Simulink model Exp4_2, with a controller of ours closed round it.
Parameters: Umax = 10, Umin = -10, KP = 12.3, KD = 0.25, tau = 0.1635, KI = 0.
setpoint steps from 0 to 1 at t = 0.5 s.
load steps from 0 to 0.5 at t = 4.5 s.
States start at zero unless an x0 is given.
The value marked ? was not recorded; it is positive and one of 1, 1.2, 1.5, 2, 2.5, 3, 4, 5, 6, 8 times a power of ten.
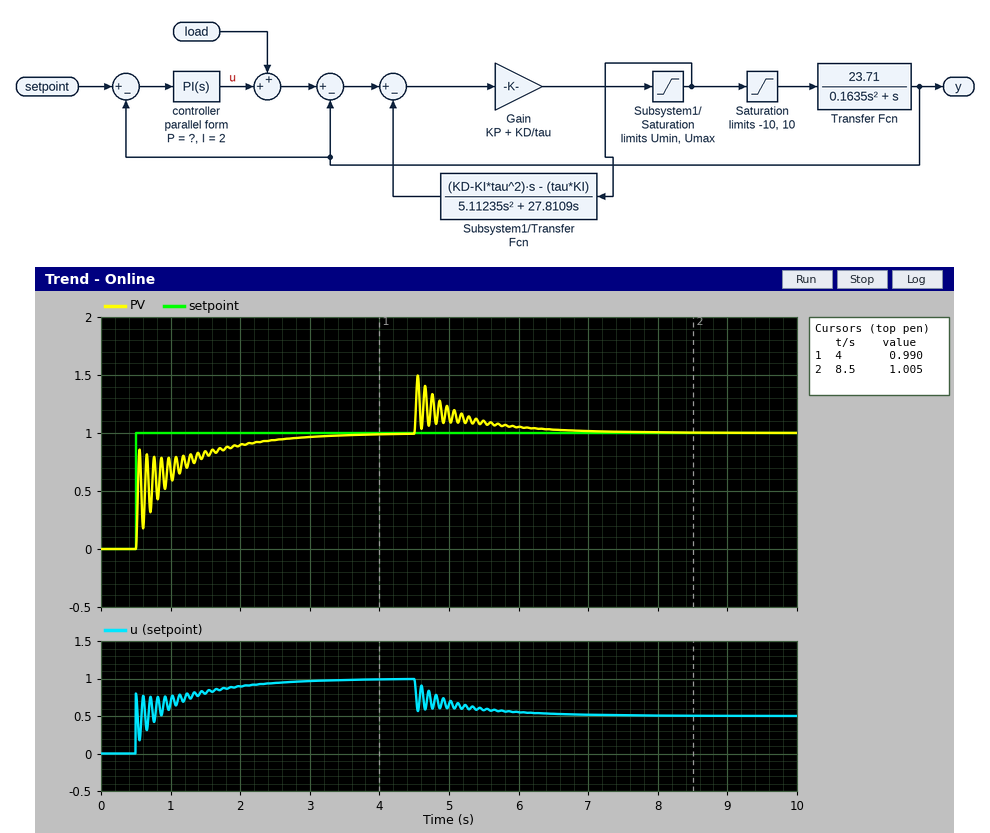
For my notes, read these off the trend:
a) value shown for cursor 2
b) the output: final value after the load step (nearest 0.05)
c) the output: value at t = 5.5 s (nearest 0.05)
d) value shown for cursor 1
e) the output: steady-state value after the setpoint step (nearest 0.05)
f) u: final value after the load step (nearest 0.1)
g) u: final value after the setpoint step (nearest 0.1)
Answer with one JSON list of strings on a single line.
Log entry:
["1.005", "1.00", "1.10", "0.990", "1.00", "0.5", "1.0"]
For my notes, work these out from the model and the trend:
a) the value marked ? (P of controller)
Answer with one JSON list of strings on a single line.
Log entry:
["0.8"]
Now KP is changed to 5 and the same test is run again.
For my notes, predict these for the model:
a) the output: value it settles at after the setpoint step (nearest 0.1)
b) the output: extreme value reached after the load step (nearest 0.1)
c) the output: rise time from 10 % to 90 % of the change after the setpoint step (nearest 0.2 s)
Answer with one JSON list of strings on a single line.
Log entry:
["1.0", "1.5", "1.6 s"]
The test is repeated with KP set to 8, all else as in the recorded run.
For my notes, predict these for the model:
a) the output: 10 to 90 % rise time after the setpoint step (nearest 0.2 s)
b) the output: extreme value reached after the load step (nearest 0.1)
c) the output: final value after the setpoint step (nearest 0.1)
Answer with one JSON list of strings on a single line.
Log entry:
["1.6 s", "1.5", "1.0"]
